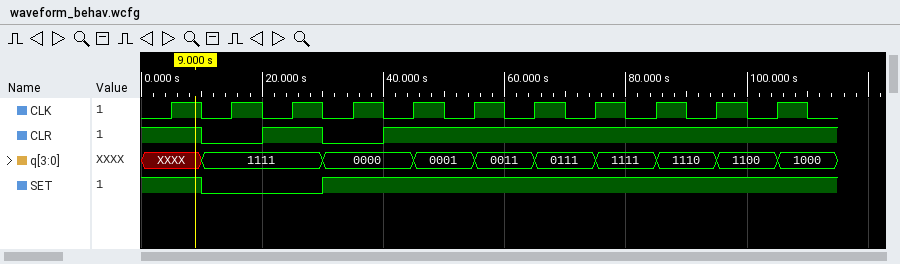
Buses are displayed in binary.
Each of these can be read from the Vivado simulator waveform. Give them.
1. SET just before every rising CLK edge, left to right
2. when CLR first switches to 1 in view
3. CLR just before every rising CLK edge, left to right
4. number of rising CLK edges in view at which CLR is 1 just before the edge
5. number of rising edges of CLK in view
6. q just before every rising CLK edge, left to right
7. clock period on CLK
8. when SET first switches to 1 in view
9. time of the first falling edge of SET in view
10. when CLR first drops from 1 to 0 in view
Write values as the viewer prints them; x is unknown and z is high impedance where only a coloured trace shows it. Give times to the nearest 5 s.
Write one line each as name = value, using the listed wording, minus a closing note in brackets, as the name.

SET just before every rising CLK edge, left to right = 1 0 0 1 1 1 1 1 1 1 1
when CLR first switches to 1 in view = 20 s
CLR just before every rising CLK edge, left to right = 1 0 1 0 1 1 1 1 1 1 1
number of rising CLK edges in view at which CLR is 1 just before the edge = 9
number of rising edges of CLK in view = 11
q just before every rising CLK edge, left to right = XXXX, 1111, 1111, 0000, 0000, 0001, 0011, 0111, 1111, 1110, 1100
clock period on CLK = 10 s
when SET first switches to 1 in view = 30 s
time of the first falling edge of SET in view = 10 s
when CLR first drops from 1 to 0 in view = 10 s
